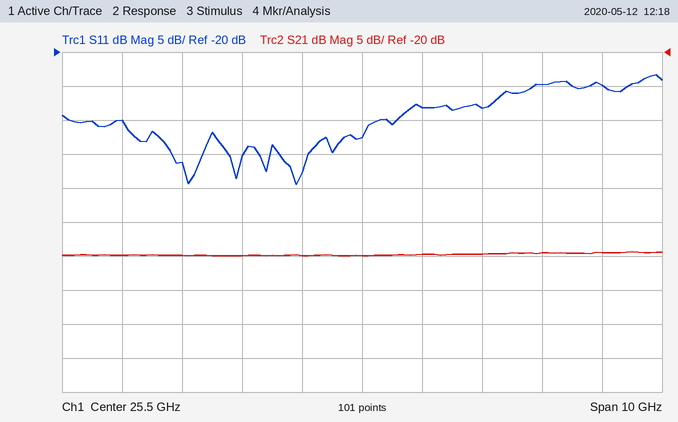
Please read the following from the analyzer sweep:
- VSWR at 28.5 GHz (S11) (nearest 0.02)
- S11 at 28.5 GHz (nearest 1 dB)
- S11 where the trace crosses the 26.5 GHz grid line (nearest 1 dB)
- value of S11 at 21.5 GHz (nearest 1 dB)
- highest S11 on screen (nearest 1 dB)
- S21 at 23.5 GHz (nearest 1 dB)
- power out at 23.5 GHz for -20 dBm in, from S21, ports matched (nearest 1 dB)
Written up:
1.12
-25 dB
-28 dB
-30 dB
-23 dB
-50 dB
-70 dBm
